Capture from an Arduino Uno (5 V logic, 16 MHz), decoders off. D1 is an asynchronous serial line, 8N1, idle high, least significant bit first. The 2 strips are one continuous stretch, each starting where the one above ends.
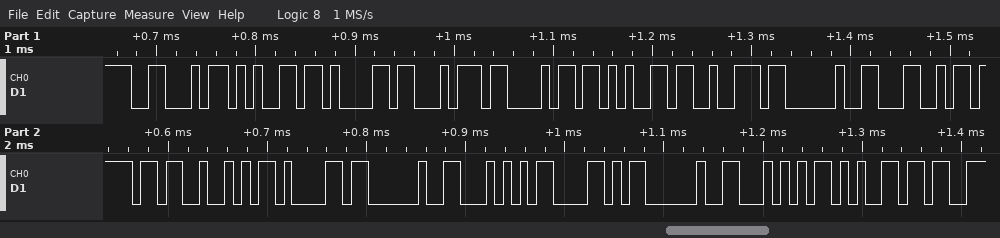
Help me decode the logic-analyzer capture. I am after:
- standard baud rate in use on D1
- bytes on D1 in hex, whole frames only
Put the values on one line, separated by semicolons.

115200 baud; 0x46 0x65 0x61 0x74 0x68 0x65 0x72 0x20 0x4C 0x6F 0x52 0x61 0x20 0x54 0x58 0x20 0x54 0x65
